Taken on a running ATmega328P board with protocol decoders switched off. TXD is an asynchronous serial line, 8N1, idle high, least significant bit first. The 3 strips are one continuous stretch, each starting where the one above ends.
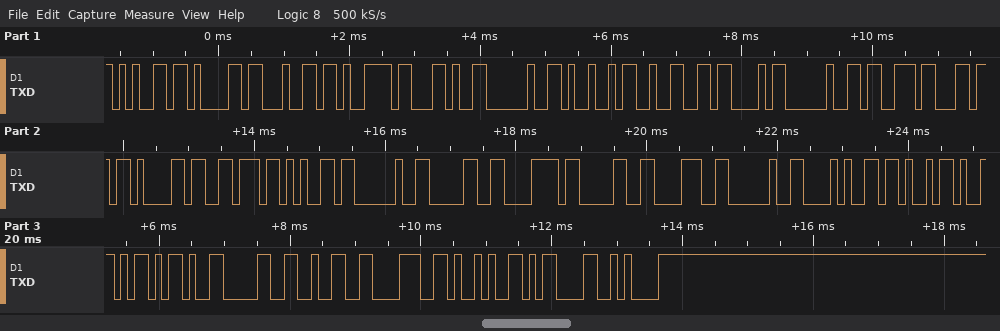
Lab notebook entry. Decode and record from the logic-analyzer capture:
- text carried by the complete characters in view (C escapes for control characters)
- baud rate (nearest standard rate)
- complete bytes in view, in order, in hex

"eady, I2C slave 0x08 (KY-028)\r\n"
9600 baud
65 61 64 79 2C 20 49 32 43 20 73 6C 61 76 65 20 30 78 30 38 20 28 4B 59 2D 30 32 38 29 0D 0A
